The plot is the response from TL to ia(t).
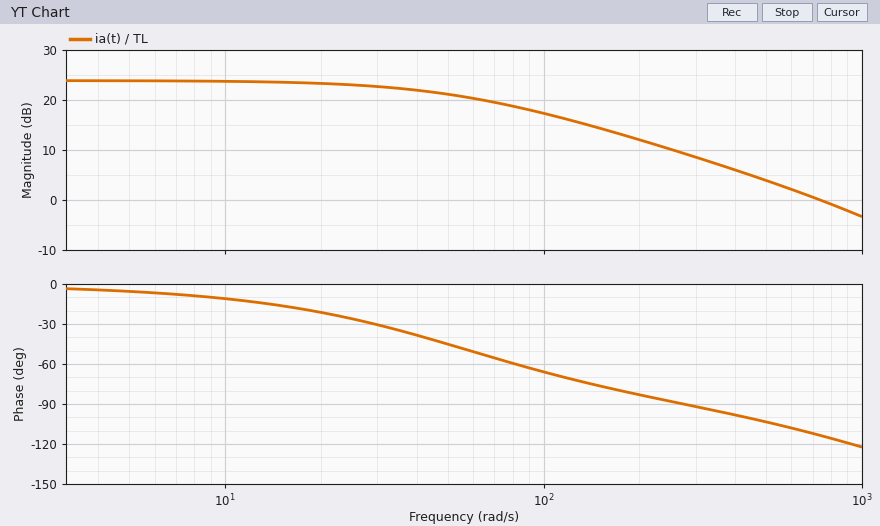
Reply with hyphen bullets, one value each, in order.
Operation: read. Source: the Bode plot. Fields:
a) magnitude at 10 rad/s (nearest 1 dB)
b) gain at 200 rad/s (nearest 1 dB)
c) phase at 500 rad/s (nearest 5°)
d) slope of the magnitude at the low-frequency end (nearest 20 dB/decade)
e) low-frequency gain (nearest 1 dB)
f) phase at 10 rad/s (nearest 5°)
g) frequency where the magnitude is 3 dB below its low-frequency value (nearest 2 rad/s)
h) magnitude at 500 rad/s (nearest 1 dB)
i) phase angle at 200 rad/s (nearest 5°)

- 24 dB
- 12 dB
- -105°
- 0 dB/decade
- 24 dB
- -10°
- 54 rad/s
- 4 dB
- -85°
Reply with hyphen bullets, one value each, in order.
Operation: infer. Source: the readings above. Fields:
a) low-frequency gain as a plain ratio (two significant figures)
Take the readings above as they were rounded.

- 16
